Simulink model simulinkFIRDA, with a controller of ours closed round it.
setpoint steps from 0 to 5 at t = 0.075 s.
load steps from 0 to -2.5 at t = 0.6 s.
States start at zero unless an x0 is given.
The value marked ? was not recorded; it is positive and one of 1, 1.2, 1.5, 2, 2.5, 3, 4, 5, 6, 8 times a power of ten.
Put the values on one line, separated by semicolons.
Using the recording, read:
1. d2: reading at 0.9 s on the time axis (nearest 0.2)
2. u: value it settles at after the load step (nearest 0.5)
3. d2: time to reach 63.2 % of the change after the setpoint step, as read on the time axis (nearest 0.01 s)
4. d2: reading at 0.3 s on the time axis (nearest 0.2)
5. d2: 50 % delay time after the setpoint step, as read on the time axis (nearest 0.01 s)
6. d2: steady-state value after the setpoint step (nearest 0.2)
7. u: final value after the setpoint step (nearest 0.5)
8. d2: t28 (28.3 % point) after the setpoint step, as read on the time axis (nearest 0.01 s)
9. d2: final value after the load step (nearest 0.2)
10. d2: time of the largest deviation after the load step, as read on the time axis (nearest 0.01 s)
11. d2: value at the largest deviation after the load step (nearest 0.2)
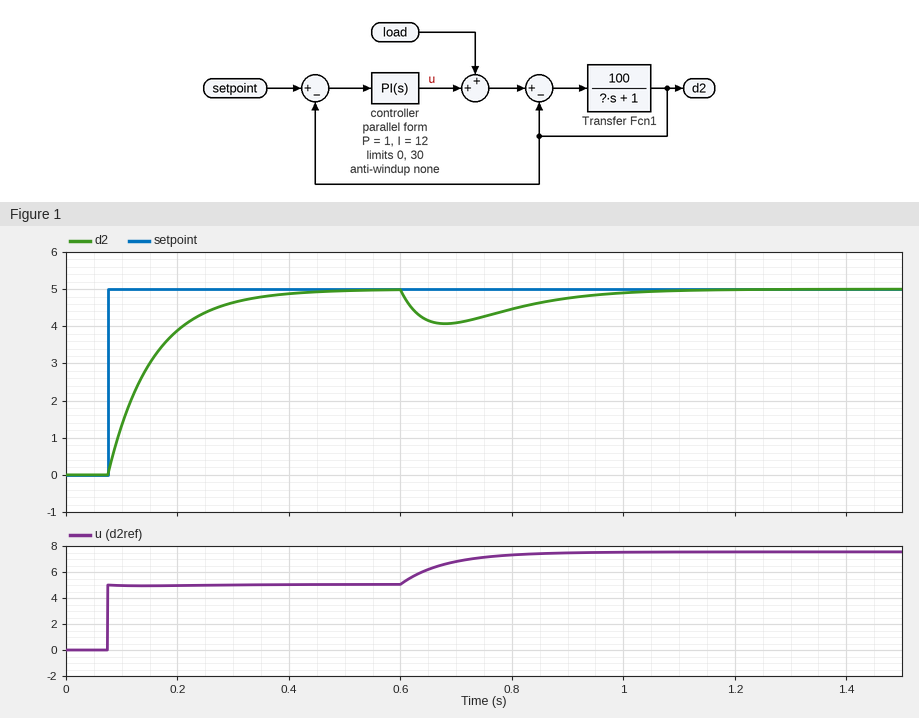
4.8; 7.5; 0.16 s; 4.6; 0.13 s; 5.0; 5.0; 0.10 s; 5.0; 0.68 s; 4.0
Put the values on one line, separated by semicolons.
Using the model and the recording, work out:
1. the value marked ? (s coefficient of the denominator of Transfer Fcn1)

8
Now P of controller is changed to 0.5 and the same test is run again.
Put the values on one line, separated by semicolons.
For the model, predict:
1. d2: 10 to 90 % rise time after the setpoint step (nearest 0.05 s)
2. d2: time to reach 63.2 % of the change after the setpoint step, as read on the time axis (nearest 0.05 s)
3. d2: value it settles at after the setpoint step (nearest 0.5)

0.15 s; 0.20 s; 5.0
